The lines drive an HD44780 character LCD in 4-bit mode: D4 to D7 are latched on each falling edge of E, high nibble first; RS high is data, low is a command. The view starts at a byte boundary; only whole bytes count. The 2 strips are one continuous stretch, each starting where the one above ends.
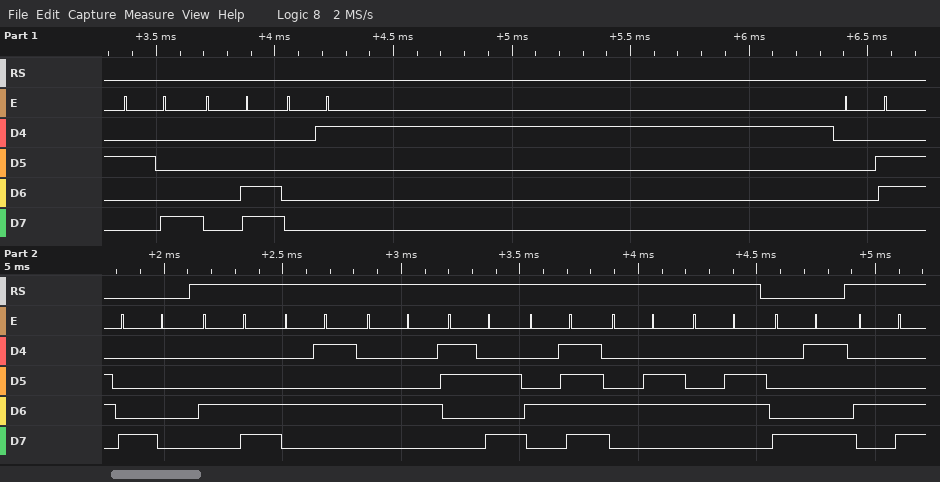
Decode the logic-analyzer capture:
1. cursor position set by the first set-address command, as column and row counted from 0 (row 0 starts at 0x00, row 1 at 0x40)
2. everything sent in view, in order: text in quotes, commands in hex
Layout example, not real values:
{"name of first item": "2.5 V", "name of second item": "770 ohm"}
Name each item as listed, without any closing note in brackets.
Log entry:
{"cursor position set by the first set-address command, as column and row counted from 0": "column 0, row 0", "everything sent in view, in order: text in quotes, commands in hex": "0x28 0x0C 0x01 0x06 0x80 \"LED:OFF\" 0x89 \"L\""}
